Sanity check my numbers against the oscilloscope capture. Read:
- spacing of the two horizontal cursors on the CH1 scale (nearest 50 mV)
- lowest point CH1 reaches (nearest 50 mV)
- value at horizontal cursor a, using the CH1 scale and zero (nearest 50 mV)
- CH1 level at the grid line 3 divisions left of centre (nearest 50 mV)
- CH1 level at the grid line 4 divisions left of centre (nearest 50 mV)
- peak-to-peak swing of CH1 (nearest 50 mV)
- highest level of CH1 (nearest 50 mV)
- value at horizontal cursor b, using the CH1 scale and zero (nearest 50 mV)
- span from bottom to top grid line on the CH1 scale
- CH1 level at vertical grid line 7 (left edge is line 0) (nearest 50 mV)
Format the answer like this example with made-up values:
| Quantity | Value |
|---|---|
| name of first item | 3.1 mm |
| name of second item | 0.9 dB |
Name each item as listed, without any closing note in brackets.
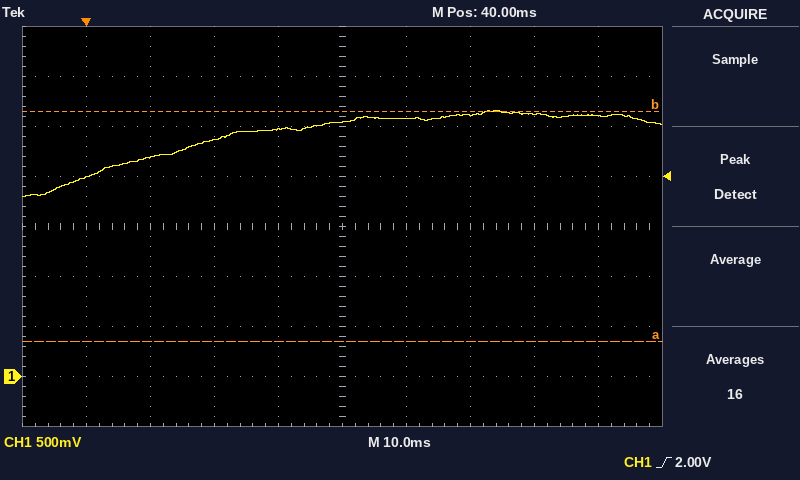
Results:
| Quantity | Value |
|---|---|
| spacing of the two horizontal cursors on the CH1 scale | 2.30 V |
| lowest point CH1 reaches | 1.80 V |
| value at horizontal cursor a, using the CH1 scale and zero | 350 mV |
| CH1 level at the grid line 3 divisions left of centre | 2.20 V |
| CH1 level at the grid line 4 divisions left of centre | 2.00 V |
| peak-to-peak swing of CH1 | 850 mV |
| highest level of CH1 | 2.65 V |
| value at horizontal cursor b, using the CH1 scale and zero | 2.65 V |
| span from bottom to top grid line on the CH1 scale | 4 V |
| CH1 level at vertical grid line 7 (left edge is line 0) | 2.60 V |
